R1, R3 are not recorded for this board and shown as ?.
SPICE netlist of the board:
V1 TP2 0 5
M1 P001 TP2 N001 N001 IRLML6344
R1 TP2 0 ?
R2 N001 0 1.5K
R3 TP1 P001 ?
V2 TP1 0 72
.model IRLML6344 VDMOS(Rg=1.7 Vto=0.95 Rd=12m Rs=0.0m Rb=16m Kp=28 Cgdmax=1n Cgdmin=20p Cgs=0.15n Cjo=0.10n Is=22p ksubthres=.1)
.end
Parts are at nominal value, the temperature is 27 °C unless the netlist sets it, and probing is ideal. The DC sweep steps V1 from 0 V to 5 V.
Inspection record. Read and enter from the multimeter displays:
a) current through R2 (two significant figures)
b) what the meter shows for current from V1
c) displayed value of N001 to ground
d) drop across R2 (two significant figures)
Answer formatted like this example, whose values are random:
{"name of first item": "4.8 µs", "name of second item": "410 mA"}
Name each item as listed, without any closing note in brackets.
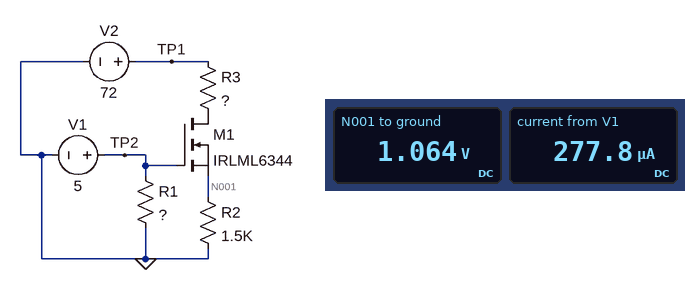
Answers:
{"current through R2": "710 µA", "what the meter shows for current from V1": "277.8 µA", "displayed value of N001 to ground": "1.064 V", "drop across R2": "1.1 V"}
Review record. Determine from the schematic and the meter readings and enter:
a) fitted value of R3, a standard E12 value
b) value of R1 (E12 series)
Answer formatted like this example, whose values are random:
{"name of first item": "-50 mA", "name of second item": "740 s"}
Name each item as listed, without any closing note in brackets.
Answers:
{"fitted value of R3, a standard E12 value": "100 kΩ", "value of R1": "18 kΩ"}
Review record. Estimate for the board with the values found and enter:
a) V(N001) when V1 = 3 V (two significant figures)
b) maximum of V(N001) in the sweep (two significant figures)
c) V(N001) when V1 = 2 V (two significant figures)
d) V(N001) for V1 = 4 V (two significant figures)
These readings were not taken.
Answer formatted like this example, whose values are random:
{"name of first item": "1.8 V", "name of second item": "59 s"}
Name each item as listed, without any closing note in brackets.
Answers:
{"V(N001) when V1 = 3 V": "1.1 V", "maximum of V(N001) in the sweep": "1.1 V", "V(N001) when V1 = 2 V": "1.1 V", "V(N001) for V1 = 4 V": "1.1 V"}
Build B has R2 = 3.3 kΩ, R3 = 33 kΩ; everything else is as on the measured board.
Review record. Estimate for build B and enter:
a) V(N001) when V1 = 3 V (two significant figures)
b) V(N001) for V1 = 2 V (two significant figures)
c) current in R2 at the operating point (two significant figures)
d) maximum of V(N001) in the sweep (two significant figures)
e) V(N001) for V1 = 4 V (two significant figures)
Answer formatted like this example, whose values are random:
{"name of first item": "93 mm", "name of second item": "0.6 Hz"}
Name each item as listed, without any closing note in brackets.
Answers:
{"V(N001) when V1 = 3 V": "2.3 V", "V(N001) for V1 = 2 V": "1.3 V", "current in R2 at the operating point": "1.3 mA", "maximum of V(N001) in the sweep": "4.3 V", "V(N001) for V1 = 4 V": "3.3 V"}
